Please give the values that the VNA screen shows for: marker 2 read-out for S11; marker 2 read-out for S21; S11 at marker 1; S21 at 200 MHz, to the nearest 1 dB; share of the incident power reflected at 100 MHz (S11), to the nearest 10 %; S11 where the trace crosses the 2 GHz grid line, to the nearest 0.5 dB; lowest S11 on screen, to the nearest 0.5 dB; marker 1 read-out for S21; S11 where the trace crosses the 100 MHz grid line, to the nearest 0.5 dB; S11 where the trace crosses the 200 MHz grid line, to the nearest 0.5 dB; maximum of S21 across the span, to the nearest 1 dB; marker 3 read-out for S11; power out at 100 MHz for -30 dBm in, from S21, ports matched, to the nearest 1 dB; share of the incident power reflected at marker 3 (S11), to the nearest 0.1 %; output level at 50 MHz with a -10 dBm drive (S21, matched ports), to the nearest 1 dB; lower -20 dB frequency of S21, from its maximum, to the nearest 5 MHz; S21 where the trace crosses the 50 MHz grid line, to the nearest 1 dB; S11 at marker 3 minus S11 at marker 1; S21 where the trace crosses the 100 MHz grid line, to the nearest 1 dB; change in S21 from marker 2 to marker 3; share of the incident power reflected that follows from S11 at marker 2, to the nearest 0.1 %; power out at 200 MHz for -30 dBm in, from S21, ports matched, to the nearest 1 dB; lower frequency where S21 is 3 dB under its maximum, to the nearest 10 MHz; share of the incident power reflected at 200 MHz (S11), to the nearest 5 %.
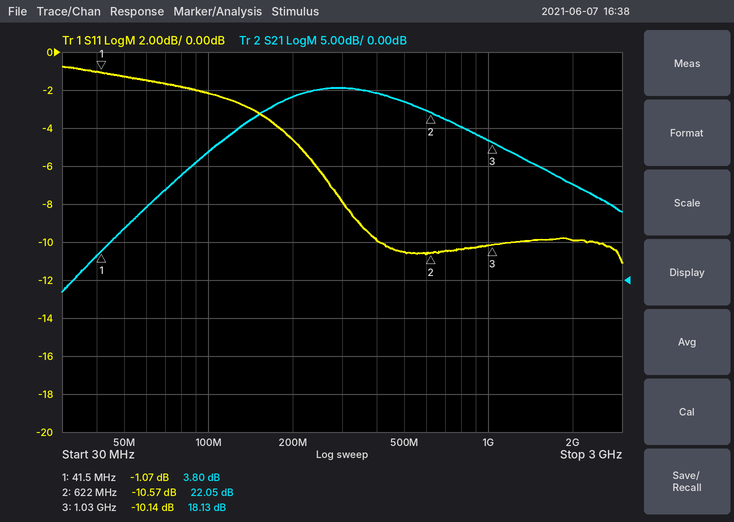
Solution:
-10.57 dB
22.05 dB
-1.07 dB
24 dB
60 %
-10.0 dB
-11.0 dB
3.80 dB
-2.0 dB
-4.5 dB
25 dB
-10.14 dB
-13 dBm
9.7 %
-3 dBm
45 MHz
7 dB
-9.07 dB
17 dB
-3.92 dB
8.8 %
-6 dBm
160 MHz
35 %
